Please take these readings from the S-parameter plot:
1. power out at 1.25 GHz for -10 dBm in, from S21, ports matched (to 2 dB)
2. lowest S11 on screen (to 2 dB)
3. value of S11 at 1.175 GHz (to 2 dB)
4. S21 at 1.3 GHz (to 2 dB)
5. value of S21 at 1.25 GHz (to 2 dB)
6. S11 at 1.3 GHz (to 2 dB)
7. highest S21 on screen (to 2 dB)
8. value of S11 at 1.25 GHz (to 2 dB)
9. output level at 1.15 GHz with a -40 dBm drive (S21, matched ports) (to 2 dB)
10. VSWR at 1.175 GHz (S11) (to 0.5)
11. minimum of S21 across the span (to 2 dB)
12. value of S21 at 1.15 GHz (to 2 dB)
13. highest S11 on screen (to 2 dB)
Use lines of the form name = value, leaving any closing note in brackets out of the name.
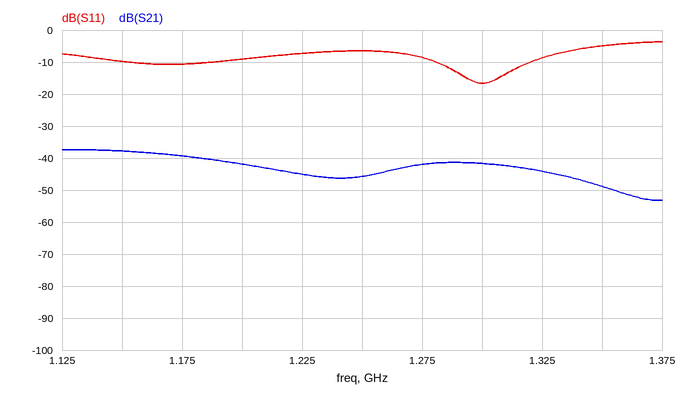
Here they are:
power out at 1.25 GHz for -10 dBm in, from S21, ports matched = -56 dBm
lowest S11 on screen = -16 dB
value of S11 at 1.175 GHz = -10 dB
S21 at 1.3 GHz = -42 dB
value of S21 at 1.25 GHz = -46 dB
S11 at 1.3 GHz = -16 dB
highest S21 on screen = -38 dB
value of S11 at 1.25 GHz = -6 dB
output level at 1.15 GHz with a -40 dBm drive (S21, matched ports) = -78 dBm
VSWR at 1.175 GHz (S11) = 2.0
minimum of S21 across the span = -54 dB
value of S21 at 1.15 GHz = -38 dB
highest S11 on screen = -4 dB
